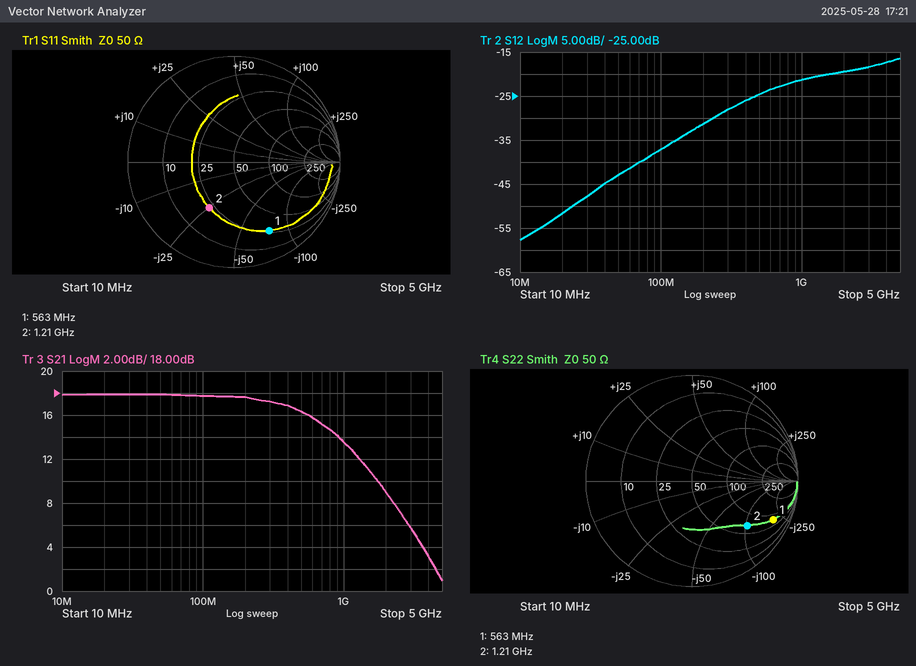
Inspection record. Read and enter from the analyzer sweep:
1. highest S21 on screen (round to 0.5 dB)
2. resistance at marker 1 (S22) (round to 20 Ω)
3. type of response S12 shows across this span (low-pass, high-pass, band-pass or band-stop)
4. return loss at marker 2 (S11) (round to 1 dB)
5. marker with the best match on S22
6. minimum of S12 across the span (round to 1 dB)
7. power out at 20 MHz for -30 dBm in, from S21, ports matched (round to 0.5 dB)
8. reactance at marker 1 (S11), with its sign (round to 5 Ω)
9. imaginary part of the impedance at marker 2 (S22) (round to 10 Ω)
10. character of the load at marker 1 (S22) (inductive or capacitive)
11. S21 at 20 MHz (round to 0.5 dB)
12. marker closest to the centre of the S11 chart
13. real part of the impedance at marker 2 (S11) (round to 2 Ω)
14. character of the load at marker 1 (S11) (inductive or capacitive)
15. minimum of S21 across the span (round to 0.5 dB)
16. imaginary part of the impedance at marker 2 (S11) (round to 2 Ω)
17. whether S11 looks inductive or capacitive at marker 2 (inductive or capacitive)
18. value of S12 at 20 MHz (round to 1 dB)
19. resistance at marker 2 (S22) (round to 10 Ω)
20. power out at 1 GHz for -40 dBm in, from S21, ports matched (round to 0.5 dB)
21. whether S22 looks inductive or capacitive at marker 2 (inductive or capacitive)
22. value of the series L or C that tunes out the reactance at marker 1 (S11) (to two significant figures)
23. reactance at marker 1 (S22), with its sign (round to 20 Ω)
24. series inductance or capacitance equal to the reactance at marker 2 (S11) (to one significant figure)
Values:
18.0 dB
80 Ω
high-pass
6 dB
marker 2
-58 dB
-12.0 dBm
-75 Ω
-100 Ω
capacitive
18.0 dB
marker 2
22 Ω
capacitive
1.0 dB
-26 Ω
capacitive
-52 dB
70 Ω
-26.5 dBm
capacitive
21 nH
-200 Ω
5 pF
